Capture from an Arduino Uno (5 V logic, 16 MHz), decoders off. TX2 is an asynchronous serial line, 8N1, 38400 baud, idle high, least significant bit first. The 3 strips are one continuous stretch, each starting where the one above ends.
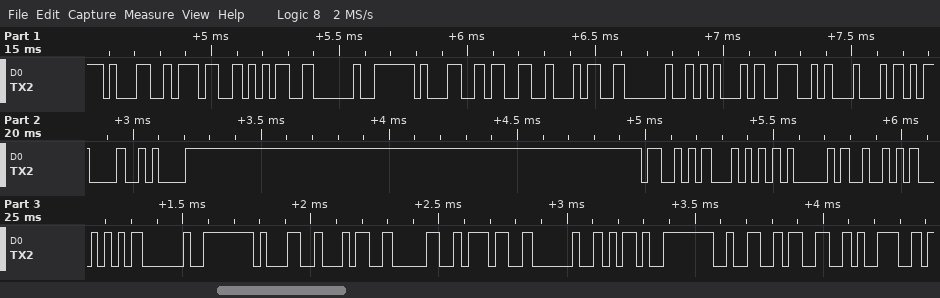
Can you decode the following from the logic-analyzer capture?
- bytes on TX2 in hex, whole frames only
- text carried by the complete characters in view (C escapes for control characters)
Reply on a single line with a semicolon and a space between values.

31 37 35 20 31 33 34 20 45 4E 44 0D 0A 53 54 41 52 54 20 31 34 30 37 20 2D 32 33 39; "175 134 END\r\nSTART 1407 -239"
